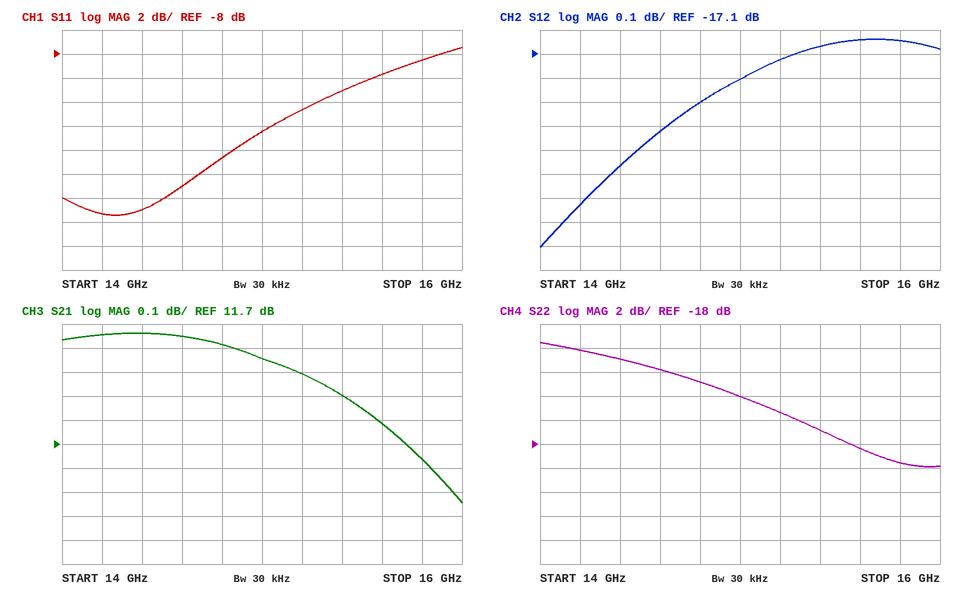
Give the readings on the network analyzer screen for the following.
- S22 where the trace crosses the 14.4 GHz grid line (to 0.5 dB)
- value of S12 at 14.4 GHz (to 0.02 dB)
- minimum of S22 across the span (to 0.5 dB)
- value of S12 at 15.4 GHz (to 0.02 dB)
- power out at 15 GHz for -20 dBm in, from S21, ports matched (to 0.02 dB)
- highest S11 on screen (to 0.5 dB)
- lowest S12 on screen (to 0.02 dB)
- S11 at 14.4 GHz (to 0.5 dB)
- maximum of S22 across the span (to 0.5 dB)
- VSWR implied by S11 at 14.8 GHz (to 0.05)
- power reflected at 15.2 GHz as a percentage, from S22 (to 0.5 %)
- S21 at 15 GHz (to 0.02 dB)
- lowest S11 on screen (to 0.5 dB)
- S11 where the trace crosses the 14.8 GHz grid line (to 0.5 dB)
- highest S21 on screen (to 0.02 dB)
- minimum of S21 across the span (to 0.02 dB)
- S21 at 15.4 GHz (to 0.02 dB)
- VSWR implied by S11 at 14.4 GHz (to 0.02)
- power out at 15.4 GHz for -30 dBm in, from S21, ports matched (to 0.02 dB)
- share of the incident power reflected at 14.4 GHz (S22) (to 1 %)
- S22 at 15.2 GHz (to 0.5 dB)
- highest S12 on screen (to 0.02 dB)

-11.0 dB
-17.56 dB
-20.0 dB
-17.06 dB
-7.94 dBm
-7.5 dB
-17.90 dB
-21.0 dB
-9.5 dB
1.35
3.0 %
12.06 dB
-21.5 dB
-16.5 dB
12.16 dB
11.46 dB
11.90 dB
1.20
-18.10 dBm
8 %
-15.5 dB
-17.04 dB
